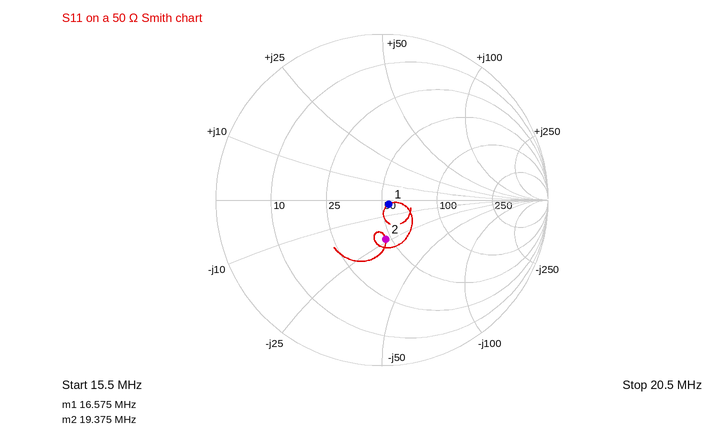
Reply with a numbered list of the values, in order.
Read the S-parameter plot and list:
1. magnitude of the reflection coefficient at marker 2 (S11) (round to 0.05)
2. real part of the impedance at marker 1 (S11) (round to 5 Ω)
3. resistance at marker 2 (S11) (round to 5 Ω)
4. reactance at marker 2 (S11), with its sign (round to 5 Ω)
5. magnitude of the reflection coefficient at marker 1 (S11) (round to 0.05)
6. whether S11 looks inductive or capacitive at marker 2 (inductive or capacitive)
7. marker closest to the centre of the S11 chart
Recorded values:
1. 0.25
2. 55 Ω
3. 45 Ω
4. -25 Ω
5. 0.05
6. capacitive
7. marker 1
